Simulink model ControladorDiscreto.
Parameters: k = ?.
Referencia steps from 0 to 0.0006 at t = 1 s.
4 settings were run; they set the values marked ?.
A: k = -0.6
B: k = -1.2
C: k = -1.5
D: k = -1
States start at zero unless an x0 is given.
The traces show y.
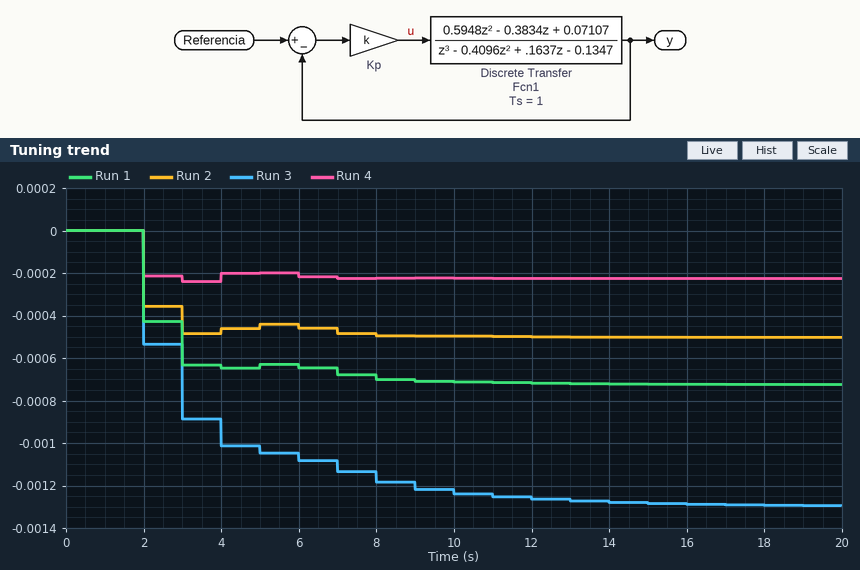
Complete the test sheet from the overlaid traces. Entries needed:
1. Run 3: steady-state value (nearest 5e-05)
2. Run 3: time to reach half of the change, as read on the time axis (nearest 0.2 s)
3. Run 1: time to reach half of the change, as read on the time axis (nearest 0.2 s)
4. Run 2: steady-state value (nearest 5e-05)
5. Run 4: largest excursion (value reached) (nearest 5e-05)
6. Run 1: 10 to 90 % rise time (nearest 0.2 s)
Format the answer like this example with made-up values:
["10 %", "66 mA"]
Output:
["-0.00130", "3.0 s", "2.0 s", "-0.00050", "-0.00025", "5.0 s"]
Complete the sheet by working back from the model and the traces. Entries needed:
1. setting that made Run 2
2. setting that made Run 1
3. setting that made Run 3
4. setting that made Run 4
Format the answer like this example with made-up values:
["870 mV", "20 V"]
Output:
["D", "B", "C", "A"]
